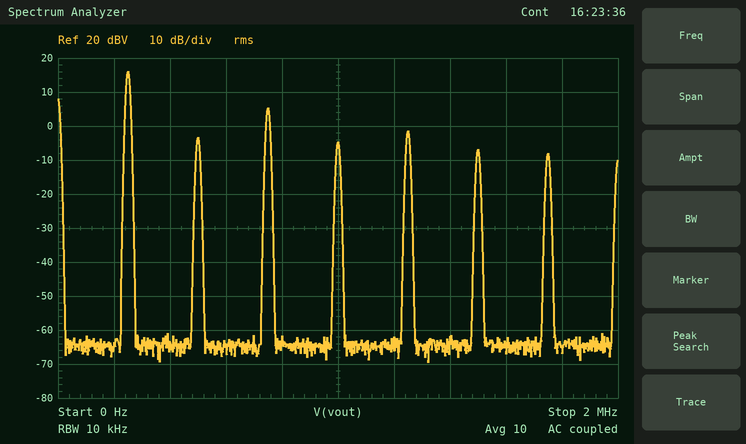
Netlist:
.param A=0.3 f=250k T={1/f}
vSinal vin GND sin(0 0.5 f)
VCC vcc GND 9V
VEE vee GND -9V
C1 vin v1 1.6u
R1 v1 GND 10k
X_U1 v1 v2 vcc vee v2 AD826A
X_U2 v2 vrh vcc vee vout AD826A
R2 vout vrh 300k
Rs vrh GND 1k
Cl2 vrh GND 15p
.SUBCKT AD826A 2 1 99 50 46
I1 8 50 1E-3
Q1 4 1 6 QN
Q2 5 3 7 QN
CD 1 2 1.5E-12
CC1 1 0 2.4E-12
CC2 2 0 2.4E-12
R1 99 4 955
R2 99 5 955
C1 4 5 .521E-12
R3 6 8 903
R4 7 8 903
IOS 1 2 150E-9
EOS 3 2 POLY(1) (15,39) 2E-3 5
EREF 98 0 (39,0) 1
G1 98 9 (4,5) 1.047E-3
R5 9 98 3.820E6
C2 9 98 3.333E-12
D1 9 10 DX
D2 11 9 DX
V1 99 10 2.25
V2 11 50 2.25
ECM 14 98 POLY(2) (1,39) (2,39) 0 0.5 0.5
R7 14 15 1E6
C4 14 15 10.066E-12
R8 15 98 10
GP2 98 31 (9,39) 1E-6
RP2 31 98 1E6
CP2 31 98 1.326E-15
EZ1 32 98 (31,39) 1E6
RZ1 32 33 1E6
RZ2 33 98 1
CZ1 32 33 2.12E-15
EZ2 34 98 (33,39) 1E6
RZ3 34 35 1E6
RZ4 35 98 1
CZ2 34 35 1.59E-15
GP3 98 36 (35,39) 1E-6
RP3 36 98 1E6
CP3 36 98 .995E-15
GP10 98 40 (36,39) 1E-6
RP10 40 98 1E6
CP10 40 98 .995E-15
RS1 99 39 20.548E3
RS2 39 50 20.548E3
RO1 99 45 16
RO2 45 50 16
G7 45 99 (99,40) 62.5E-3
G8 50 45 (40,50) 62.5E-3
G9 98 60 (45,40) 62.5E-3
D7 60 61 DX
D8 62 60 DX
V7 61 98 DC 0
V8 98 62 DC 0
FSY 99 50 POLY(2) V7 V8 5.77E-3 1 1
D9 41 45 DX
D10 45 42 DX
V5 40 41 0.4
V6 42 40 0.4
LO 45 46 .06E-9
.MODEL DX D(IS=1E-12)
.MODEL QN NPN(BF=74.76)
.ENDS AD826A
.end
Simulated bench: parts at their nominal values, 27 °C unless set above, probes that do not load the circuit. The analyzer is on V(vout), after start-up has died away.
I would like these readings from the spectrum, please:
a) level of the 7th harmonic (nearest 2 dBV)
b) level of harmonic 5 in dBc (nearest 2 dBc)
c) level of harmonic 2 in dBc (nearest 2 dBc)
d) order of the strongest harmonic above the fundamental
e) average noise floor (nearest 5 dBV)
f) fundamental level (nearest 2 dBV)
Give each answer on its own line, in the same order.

-8 dBV
-18 dBc
-20 dBc
3
-65 dBV
16 dBV
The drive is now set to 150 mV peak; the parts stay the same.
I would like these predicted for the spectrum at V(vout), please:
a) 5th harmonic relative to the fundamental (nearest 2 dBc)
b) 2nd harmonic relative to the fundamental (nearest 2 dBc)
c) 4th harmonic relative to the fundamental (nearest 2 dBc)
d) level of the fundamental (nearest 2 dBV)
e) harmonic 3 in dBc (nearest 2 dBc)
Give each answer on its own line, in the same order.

-30 dBc
-10 dBc
-18 dBc
16 dBV
-20 dBc
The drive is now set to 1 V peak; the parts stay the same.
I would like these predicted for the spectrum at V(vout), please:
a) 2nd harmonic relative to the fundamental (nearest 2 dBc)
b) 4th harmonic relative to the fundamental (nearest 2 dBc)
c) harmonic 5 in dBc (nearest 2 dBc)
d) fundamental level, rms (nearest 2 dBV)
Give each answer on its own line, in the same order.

-26 dBc
-26 dBc
-16 dBc
16 dBV
